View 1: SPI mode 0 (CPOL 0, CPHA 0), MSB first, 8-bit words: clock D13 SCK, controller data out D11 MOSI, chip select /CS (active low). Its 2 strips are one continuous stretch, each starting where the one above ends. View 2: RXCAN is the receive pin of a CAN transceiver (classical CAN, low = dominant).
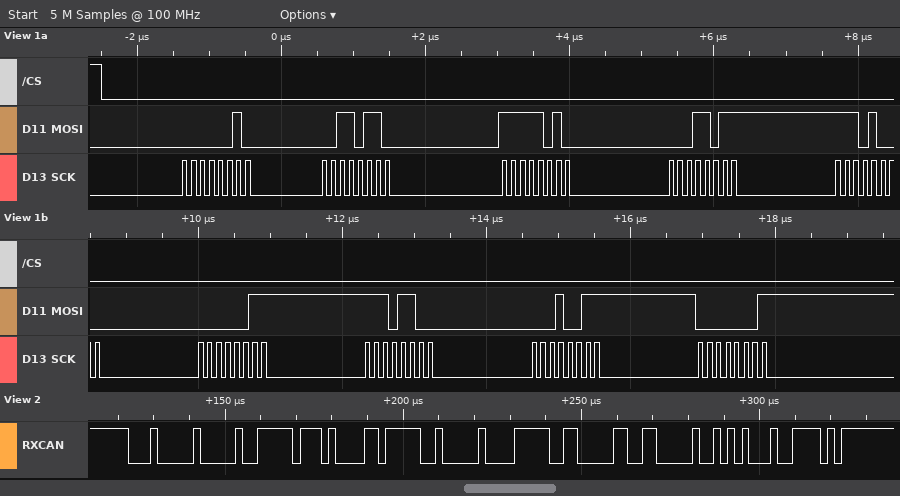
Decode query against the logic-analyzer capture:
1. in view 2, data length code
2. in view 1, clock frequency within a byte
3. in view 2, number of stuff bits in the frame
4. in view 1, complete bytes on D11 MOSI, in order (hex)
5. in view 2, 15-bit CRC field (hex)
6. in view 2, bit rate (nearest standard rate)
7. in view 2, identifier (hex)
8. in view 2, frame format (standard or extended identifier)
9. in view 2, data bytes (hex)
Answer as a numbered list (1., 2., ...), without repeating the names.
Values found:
1. 7
2. 8 MHz
3. 8
4. 02 36 FA 1B E8 03 EC 13 01
5. 0x289E
6. 500 kbit/s
7. 0x100
8. standard
9. FA 1B E8 03 EC 13 01
